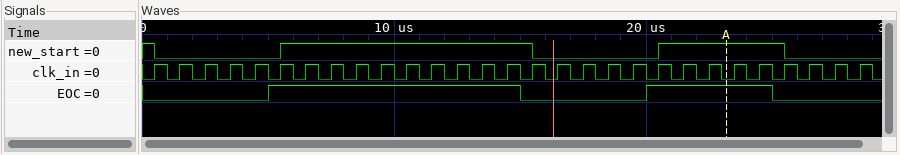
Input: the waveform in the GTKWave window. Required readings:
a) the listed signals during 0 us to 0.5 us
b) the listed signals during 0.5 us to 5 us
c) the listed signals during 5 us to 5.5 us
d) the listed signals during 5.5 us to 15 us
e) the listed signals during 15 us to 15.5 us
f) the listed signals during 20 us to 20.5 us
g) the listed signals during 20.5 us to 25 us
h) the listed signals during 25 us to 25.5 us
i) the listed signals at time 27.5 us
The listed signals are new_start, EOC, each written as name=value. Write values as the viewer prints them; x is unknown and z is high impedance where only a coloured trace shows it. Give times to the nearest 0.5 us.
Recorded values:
new_start=1, EOC=0
new_start=0, EOC=0
new_start=0, EOC=1
new_start=1, EOC=1
new_start=1, EOC=0
new_start=0, EOC=1
new_start=1, EOC=1
new_start=1, EOC=0
new_start=0, EOC=0
